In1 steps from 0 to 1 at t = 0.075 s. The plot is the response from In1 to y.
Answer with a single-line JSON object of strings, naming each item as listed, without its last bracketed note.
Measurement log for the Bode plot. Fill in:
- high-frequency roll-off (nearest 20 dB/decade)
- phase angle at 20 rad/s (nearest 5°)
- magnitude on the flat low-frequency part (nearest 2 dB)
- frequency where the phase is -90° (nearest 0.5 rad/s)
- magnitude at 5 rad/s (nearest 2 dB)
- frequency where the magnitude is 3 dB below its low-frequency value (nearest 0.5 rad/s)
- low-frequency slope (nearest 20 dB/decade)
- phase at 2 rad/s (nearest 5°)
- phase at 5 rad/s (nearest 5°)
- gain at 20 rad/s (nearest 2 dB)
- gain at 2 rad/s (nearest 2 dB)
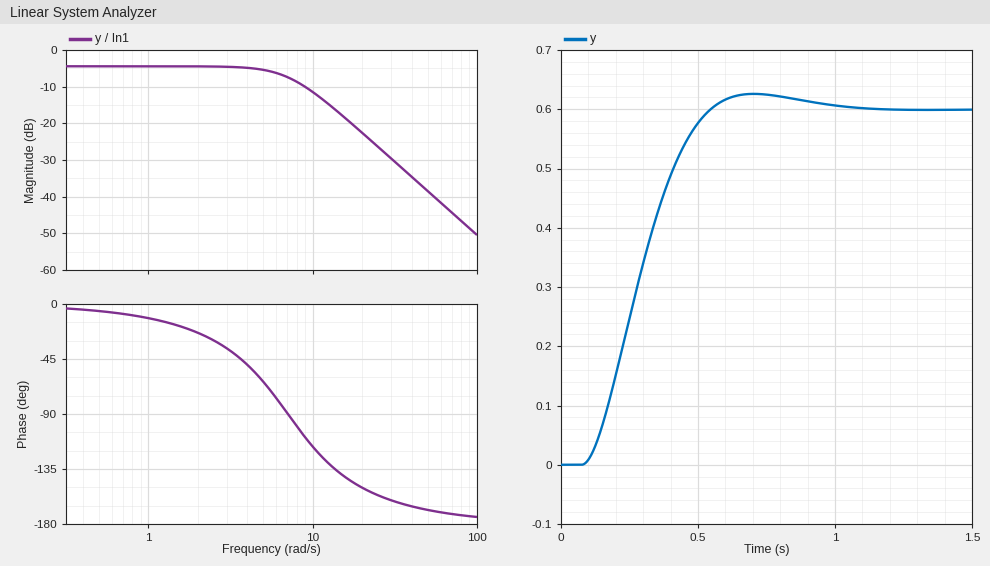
{"high-frequency roll-off": "-40 dB/decade", "phase angle at 20 rad/s": "-150°", "magnitude on the flat low-frequency part": "-4 dB", "frequency where the phase is -90°": "7.0 rad/s", "magnitude at 5 rad/s": "-6 dB", "frequency where the magnitude is 3 dB below its low-frequency value": "7.0 rad/s", "low-frequency slope": "0 dB/decade", "phase at 2 rad/s": "-25°", "phase at 5 rad/s": "-65°", "gain at 20 rad/s": "-22 dB", "gain at 2 rad/s": "-4 dB"}
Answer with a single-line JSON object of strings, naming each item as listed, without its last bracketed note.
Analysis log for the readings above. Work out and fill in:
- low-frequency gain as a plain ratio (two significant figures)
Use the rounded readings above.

{"low-frequency gain as a plain ratio": "0.63"}
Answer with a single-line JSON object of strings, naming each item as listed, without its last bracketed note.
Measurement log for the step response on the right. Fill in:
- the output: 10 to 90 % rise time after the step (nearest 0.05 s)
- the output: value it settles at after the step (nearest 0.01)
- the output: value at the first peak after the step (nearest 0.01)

{"the output: 10 to 90 % rise time after the step": "0.30 s", "the output: value it settles at after the step": "0.60", "the output: value at the first peak after the step": "0.63"}
